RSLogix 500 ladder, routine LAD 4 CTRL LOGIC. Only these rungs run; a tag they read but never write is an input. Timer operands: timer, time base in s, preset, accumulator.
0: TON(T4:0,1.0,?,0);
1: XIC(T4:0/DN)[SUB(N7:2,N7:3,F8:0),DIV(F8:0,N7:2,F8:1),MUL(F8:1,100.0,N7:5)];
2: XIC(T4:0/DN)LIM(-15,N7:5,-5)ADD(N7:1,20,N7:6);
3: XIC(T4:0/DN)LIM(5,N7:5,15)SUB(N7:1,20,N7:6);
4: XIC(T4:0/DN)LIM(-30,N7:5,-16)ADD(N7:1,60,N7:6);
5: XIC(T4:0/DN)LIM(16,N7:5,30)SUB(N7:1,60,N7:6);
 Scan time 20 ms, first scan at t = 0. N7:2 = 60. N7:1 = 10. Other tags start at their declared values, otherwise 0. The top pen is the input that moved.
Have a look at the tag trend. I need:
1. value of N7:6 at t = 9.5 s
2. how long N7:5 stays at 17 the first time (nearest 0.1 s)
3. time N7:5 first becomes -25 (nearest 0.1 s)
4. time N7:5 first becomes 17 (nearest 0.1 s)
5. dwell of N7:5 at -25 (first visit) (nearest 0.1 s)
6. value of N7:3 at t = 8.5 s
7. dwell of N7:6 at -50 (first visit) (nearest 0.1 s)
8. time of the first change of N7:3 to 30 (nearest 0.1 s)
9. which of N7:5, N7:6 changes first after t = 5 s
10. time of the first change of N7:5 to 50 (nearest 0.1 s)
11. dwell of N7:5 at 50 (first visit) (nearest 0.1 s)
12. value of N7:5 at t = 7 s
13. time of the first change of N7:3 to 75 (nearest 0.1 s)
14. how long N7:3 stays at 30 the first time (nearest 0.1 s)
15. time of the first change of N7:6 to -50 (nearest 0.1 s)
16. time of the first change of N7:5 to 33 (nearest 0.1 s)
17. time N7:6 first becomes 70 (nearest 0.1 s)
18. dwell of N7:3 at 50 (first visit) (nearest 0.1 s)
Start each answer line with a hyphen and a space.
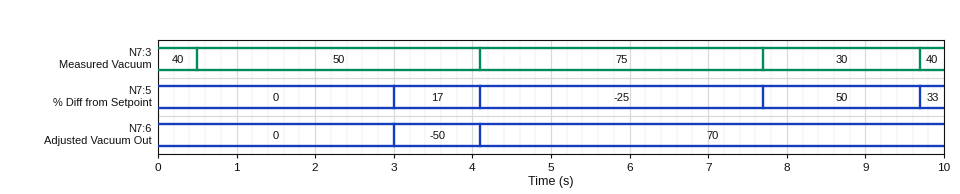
- 70
- 1.1 s
- 4.1 s
- 3.0 s
- 3.6 s
- 30
- 1.1 s
- 7.7 s
- N7:5
- 7.7 s
- 2.0 s
- -25
- 4.1 s
- 2.0 s
- 3.0 s
- 9.7 s
- 4.1 s
- 3.6 s
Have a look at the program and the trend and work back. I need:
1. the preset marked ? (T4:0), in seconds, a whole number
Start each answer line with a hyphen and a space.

- 3 s
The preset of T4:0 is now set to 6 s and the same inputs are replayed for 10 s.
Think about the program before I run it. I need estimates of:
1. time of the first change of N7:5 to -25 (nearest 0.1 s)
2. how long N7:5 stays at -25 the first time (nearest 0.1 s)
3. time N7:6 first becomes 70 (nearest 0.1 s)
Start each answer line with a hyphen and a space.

- 6.0 s
- 1.7 s
- 6.0 s
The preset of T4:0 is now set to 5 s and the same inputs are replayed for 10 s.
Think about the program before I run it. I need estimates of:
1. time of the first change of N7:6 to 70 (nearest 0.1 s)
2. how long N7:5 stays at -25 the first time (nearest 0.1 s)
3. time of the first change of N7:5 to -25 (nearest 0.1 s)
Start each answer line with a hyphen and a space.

- 5.0 s
- 2.7 s
- 5.0 s
